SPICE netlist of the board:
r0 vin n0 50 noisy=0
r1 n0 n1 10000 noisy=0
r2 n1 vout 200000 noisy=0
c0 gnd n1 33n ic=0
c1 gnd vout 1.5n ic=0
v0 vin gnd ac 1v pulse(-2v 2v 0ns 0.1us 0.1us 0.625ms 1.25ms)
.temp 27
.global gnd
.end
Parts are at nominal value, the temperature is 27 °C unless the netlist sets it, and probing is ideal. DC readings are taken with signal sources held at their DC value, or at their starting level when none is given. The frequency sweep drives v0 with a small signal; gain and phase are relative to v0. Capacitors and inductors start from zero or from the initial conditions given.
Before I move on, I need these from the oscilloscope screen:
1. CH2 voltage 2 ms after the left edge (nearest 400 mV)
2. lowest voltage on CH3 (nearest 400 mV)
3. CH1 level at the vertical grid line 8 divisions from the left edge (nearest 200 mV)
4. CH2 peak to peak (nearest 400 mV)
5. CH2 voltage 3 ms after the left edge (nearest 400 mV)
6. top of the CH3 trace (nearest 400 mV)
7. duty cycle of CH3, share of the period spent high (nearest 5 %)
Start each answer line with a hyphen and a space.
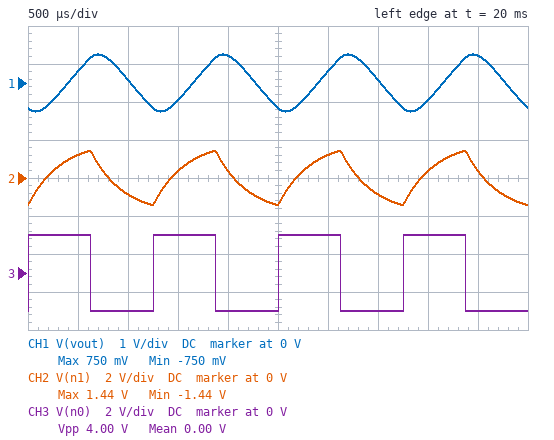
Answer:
- 400 mV
- -2.0 V
- -400 mV
- 2.8 V
- 1.2 V
- 2.0 V
- 50 %
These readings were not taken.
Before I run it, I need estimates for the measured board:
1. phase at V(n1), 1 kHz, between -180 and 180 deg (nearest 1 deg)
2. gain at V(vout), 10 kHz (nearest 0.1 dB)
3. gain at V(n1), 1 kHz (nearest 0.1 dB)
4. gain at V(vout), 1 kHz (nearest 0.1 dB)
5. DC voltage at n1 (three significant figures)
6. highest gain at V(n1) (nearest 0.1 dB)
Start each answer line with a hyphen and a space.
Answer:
- -64 deg
- -51.9 dB
- -7.4 dB
- -14.0 dB
- -2.00 V
- 0 dB
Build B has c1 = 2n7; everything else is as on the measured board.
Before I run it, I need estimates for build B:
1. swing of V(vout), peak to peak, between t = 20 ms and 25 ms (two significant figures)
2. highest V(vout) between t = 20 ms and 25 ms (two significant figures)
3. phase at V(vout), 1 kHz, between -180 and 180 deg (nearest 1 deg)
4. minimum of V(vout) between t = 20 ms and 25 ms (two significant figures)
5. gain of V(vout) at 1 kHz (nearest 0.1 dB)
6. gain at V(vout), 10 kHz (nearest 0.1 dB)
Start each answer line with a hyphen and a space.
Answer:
- 920 mV
- 460 mV
- -137 deg
- -460 mV
- -18.4 dB
- -57.0 dB
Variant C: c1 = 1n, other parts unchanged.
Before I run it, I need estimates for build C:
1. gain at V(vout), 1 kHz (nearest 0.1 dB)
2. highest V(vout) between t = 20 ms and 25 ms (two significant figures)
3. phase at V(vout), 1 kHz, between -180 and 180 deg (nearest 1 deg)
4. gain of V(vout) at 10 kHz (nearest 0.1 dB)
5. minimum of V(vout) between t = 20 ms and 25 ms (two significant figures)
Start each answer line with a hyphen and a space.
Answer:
- -11.5 dB
- 970 mV
- -115 deg
- -48.4 dB
- -970 mV
